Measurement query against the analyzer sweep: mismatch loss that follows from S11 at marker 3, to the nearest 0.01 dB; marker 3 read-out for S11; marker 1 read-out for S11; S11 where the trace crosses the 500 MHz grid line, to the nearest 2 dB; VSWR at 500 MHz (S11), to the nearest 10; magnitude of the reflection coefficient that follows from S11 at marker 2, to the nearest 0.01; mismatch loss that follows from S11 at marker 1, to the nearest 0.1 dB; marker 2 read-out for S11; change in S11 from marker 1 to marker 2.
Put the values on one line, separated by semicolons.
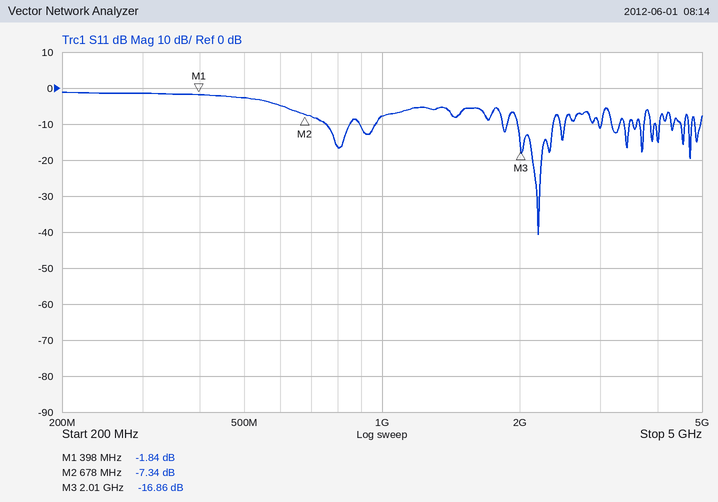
0.09 dB; -16.86 dB; -1.84 dB; -2 dB; 10; 0.43; 4.6 dB; -7.34 dB; -5.50 dB
